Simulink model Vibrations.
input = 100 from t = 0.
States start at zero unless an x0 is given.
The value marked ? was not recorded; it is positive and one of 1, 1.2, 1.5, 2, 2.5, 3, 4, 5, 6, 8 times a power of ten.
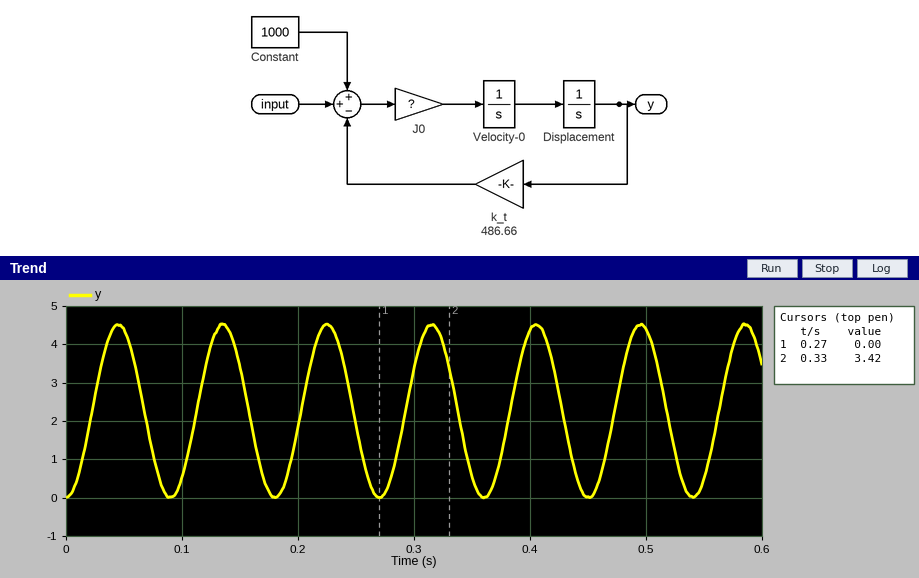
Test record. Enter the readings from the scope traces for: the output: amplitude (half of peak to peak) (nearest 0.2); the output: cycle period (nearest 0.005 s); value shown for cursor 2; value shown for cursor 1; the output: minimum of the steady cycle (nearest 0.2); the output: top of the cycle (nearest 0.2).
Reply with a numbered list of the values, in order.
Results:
1. 2.2
2. 0.090 s
3. 3.42
4. 0.00
5. 0.0
6. 4.6
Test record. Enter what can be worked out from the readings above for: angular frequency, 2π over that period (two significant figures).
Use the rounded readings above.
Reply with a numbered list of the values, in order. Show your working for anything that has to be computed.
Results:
1. 2π / 0.09 = 70 rad/s
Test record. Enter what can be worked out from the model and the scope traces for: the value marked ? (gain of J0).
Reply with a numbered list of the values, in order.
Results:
1. 10
